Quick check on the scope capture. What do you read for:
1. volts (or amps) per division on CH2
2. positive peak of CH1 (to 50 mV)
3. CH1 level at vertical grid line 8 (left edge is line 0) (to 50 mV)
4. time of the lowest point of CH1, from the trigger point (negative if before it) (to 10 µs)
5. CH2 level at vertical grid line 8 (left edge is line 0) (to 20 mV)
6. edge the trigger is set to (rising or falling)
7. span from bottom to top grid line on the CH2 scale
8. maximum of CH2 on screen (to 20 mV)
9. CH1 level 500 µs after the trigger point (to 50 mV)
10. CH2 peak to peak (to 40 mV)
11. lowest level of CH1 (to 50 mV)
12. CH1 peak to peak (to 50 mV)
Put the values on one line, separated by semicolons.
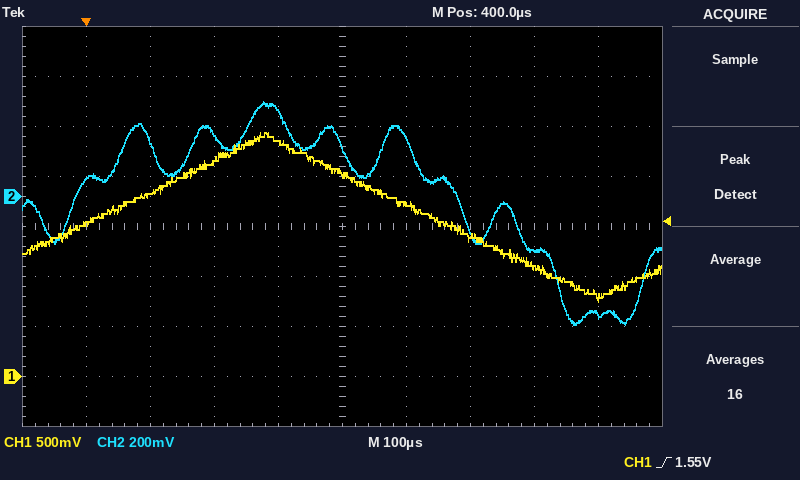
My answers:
200 mV; 2.45 V; 1.10 V; +800 µs; -220 mV; rising; 1.6 V; 380 mV; 1.75 V; 880 mV; 750 mV; 1.70 V
